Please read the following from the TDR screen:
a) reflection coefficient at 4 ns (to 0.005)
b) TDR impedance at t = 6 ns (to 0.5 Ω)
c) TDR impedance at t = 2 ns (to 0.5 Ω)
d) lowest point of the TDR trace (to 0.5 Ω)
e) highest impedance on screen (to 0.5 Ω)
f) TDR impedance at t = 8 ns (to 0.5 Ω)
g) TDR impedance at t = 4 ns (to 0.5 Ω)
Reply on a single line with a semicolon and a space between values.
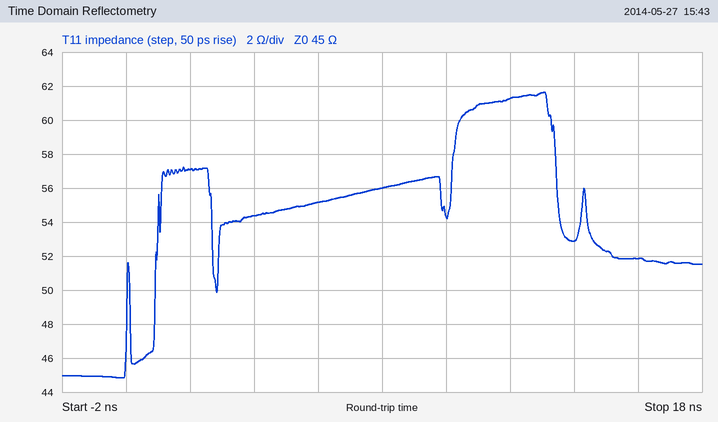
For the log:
+0.095; 55.0 Ω; 57.0 Ω; 45.0 Ω; 61.5 Ω; 56.0 Ω; 54.5 Ω
